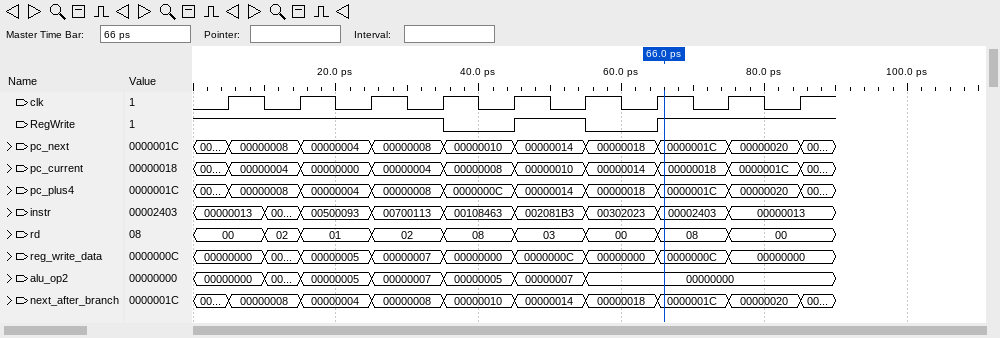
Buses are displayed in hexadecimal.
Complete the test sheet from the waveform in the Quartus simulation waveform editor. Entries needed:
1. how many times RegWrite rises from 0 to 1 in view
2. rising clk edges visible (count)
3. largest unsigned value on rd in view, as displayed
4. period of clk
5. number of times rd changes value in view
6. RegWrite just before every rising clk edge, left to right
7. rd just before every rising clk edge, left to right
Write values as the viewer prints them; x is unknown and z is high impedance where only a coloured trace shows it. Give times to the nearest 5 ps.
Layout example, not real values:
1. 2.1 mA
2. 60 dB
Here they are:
1. 2
2. 9
3. 08
4. 10 ps
5. 8
6. 1 1 1 1 0 1 0 1 1
7. 00, 02, 01, 02, 08, 03, 00, 08, 00
